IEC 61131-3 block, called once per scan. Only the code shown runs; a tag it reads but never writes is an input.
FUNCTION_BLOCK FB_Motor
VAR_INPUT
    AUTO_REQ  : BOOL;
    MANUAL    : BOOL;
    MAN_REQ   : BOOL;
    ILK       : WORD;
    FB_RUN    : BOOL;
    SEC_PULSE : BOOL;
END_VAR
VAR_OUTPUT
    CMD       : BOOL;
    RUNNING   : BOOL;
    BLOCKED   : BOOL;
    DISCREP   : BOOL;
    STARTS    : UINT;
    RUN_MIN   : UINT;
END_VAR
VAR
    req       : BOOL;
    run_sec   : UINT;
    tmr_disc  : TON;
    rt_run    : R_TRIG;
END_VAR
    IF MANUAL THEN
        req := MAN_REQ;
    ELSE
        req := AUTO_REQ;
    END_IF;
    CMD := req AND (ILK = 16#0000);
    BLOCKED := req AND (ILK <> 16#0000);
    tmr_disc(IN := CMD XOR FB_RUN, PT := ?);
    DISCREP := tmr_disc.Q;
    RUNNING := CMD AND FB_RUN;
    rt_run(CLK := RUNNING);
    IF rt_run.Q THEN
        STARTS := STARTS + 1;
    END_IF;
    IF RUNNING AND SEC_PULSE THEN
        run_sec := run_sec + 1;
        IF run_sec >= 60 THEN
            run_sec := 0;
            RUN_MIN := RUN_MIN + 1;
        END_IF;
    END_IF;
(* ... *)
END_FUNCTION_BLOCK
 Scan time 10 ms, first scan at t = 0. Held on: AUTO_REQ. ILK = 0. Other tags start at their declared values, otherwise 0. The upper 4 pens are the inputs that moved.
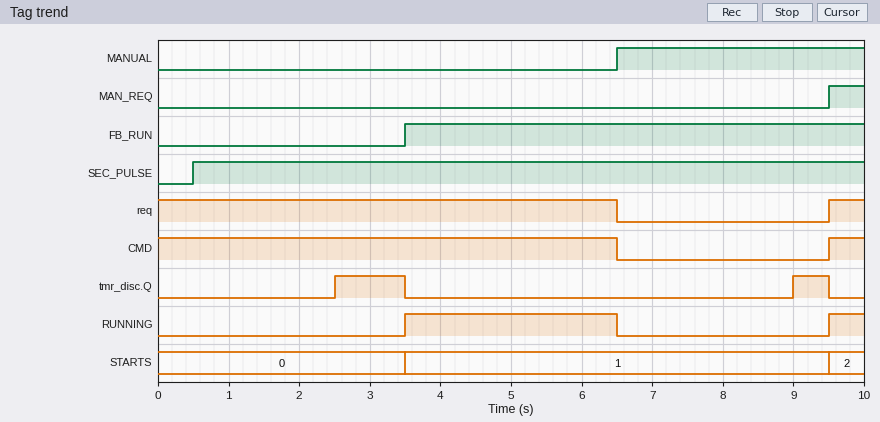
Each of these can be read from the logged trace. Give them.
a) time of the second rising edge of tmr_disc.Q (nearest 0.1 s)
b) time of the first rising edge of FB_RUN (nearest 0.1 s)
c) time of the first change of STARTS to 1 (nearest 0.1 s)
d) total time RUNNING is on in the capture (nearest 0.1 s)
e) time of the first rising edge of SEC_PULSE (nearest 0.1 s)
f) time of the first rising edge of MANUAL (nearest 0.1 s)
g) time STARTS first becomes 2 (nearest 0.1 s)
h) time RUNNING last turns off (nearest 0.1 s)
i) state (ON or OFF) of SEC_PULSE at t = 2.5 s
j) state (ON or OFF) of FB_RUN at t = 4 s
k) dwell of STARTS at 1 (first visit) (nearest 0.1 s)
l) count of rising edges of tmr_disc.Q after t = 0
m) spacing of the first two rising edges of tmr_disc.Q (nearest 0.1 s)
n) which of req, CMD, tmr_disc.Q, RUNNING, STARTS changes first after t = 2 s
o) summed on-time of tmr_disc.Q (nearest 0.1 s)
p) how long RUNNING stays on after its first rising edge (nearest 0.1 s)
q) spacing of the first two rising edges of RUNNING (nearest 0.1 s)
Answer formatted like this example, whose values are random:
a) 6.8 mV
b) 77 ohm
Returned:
a) 9.0 s
b) 3.5 s
c) 3.5 s
d) 3.5 s
e) 0.5 s
f) 6.5 s
g) 9.5 s
h) 6.5 s
i) ON
j) ON
k) 6.0 s
l) 2
m) 6.5 s
n) tmr_disc.Q
o) 1.5 s
p) 3.0 s
q) 6.0 s
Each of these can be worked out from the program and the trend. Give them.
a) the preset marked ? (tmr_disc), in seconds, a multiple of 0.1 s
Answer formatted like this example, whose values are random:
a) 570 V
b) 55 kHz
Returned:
a) 2.5 s
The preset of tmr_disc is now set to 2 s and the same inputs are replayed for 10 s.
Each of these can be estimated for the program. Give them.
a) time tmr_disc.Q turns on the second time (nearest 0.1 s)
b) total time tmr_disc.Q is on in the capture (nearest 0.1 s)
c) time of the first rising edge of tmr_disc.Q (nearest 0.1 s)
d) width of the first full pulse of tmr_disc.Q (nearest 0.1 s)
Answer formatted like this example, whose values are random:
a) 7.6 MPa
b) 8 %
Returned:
a) 8.5 s
b) 2.5 s
c) 2.0 s
d) 1.5 s
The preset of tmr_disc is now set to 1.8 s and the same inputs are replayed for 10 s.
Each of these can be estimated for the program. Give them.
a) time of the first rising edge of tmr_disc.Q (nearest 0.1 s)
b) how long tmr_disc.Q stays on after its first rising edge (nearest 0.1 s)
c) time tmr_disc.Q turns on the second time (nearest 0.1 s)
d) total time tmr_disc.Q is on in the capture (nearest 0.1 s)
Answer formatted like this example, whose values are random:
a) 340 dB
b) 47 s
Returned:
a) 1.8 s
b) 1.7 s
c) 8.3 s
d) 2.9 s
